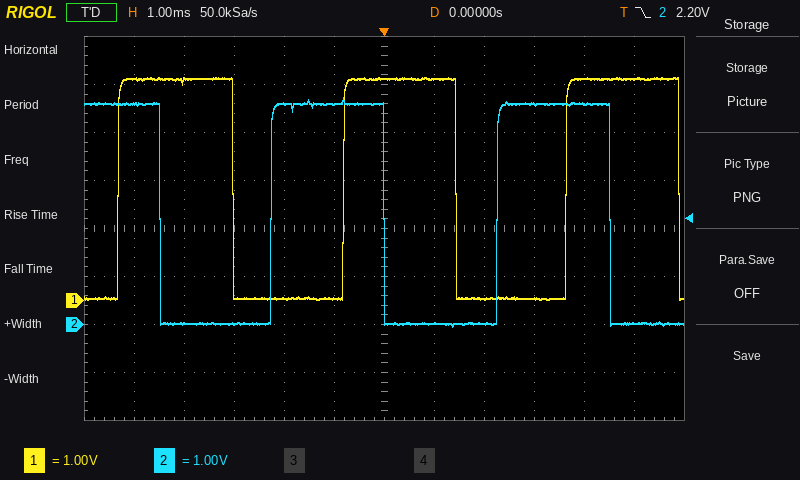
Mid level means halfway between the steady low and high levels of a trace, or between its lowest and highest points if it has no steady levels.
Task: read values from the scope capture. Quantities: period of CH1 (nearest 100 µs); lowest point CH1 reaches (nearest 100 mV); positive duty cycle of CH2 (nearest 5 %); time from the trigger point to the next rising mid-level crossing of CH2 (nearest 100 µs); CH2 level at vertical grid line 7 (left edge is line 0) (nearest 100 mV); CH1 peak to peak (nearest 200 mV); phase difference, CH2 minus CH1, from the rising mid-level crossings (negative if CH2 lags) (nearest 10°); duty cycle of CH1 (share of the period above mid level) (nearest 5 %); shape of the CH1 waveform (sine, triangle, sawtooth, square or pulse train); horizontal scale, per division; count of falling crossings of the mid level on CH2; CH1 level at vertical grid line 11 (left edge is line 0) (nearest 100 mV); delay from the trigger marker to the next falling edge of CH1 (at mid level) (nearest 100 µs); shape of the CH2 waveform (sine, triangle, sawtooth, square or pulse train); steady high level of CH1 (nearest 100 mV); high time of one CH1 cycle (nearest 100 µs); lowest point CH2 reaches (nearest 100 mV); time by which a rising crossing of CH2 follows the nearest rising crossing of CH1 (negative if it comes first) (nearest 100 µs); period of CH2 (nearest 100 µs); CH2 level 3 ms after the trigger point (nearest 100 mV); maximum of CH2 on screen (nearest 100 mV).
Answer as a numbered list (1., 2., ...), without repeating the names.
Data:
1. 4.5 ms
2. 0.0 V
3. 50 %
4. 2.3 ms
5. 0.0 V
6. 4.6 V
7. +110°
8. 50 %
9. square
10. 1 ms
11. 3
12. 4.6 V
13. 1.4 ms
14. square
15. 4.6 V
16. 2.3 ms
17. 0.0 V
18. -1.4 ms
19. 4.5 ms
20. 4.6 V
21. 4.7 V
